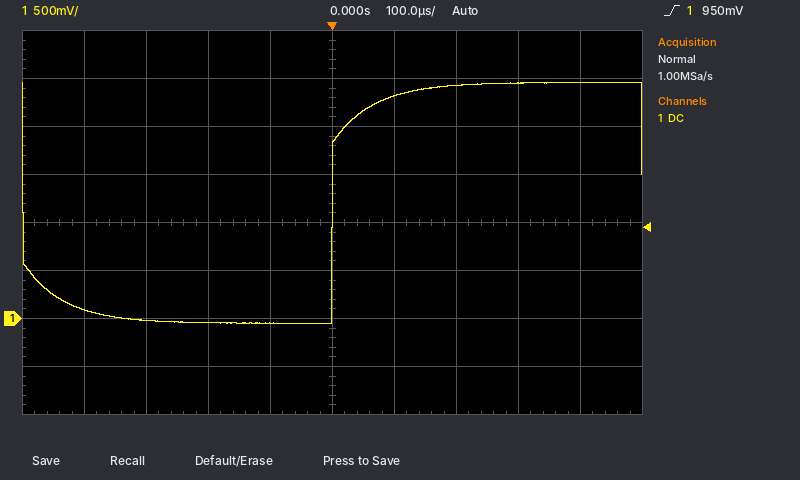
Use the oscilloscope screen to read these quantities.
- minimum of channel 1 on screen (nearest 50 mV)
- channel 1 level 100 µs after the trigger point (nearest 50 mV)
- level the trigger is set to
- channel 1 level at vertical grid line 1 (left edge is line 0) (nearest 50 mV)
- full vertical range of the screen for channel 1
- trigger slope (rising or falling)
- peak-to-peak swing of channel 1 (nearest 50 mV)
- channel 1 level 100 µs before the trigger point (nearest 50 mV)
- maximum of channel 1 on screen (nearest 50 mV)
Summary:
-50 mV
2.30 V
950 mV
100 mV
4 V
rising
2.50 V
-50 mV
2.45 V
